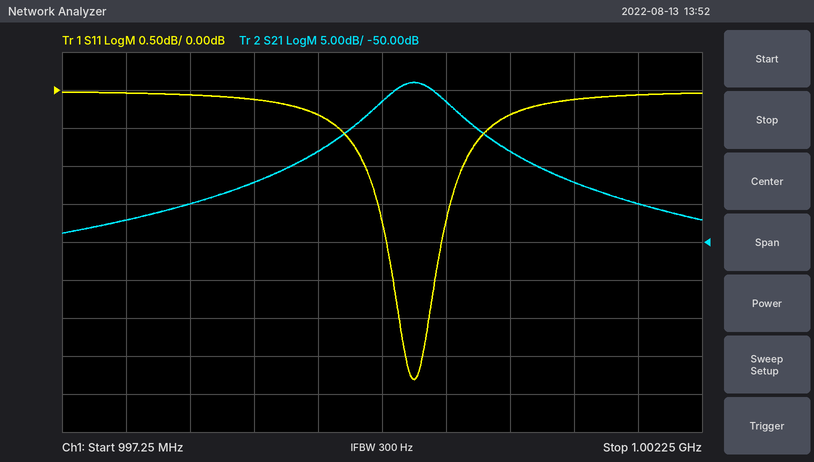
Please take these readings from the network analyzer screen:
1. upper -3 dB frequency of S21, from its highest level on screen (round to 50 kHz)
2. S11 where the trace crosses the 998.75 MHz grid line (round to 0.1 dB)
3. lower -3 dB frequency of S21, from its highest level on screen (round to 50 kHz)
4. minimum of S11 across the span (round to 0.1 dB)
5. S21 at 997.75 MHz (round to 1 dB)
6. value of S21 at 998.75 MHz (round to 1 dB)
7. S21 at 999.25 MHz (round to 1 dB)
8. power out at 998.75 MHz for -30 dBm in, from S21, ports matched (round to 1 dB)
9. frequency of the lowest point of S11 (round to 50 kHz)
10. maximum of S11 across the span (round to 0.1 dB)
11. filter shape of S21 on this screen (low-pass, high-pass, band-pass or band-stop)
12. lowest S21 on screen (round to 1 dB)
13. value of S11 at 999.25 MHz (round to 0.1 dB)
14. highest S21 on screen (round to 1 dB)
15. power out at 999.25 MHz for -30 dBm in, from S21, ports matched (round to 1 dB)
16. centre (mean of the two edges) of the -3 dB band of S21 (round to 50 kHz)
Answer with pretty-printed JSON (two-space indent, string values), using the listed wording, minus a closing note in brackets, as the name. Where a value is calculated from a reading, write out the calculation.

{
  "upper -3 dB frequency of S21, from its highest level on screen": "1.00030 GHz",
  "S11 where the trace crosses the 998.75 MHz grid line": "-0.1 dB",
  "lower -3 dB frequency of S21, from its highest level on screen": "999.70 MHz",
  "minimum of S11 across the span": "-3.8 dB",
  "S21 at 997.75 MHz": "-47 dB",
  "value of S21 at 998.75 MHz": "-42 dB",
  "S21 at 999.25 MHz": "-38 dB",
  "power out at 998.75 MHz for -30 dBm in, from S21, ports matched": "-30 dBm + (-42 dB) = -72 dBm",
  "frequency of the lowest point of S11": "1.00000 GHz",
  "maximum of S11 across the span": "0.0 dB",
  "filter shape of S21 on this screen": "band-pass",
  "lowest S21 on screen": "-49 dB",
  "value of S11 at 999.25 MHz": "-0.3 dB",
  "highest S21 on screen": "-29 dB",
  "power out at 999.25 MHz for -30 dBm in, from S21, ports matched": "-30 dBm + (-38 dB) = -68 dBm",
  "centre (mean of the two edges) of the -3 dB band of S21": "1.00000 GHz"
}
